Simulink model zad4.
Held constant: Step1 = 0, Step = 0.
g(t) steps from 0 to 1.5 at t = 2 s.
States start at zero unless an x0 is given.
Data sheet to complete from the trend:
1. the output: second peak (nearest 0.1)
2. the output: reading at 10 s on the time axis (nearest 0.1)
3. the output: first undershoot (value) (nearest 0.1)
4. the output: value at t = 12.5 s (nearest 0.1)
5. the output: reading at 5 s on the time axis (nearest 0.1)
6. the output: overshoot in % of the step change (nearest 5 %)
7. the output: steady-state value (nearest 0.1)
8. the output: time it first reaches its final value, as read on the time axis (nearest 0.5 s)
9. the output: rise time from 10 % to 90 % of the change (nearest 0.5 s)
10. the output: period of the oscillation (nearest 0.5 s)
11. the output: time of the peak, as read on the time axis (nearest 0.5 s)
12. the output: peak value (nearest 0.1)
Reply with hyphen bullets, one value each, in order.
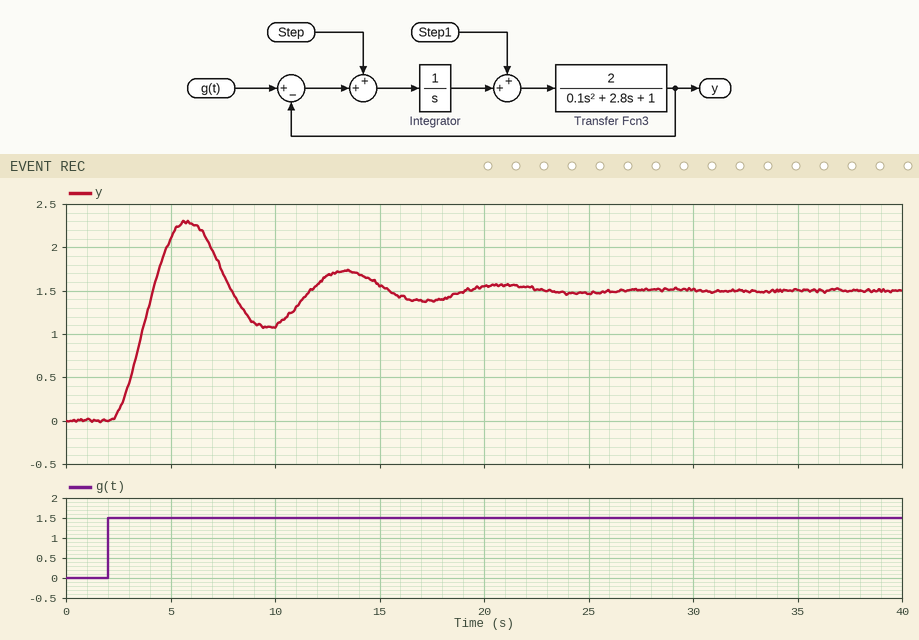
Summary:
- 1.7
- 1.1
- 1.1
- 1.7
- 2.1
- 55 %
- 1.5
- 4.0 s
- 1.5 s
- 7.5 s
- 6.0 s
- 2.3
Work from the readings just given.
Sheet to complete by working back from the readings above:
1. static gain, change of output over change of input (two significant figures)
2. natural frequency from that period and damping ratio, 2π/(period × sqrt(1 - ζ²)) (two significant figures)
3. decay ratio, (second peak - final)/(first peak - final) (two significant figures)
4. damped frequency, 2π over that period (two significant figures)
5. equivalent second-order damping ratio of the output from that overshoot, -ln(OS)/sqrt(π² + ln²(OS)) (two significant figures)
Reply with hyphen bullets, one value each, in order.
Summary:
- 1.0
- 0.85 rad/s
- 0.25
- 0.84 rad/s
- 0.19
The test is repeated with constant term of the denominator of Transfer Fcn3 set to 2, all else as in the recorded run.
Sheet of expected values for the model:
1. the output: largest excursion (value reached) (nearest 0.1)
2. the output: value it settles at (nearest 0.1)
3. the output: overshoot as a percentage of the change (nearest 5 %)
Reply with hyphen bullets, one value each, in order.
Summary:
- 1.9
- 1.5
- 25 %
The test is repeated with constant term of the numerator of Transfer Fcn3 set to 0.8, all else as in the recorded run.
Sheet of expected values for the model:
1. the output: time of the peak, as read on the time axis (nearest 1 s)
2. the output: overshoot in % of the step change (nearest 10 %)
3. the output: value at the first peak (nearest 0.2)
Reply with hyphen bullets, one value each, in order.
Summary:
- 8 s
- 30 %
- 2.0
